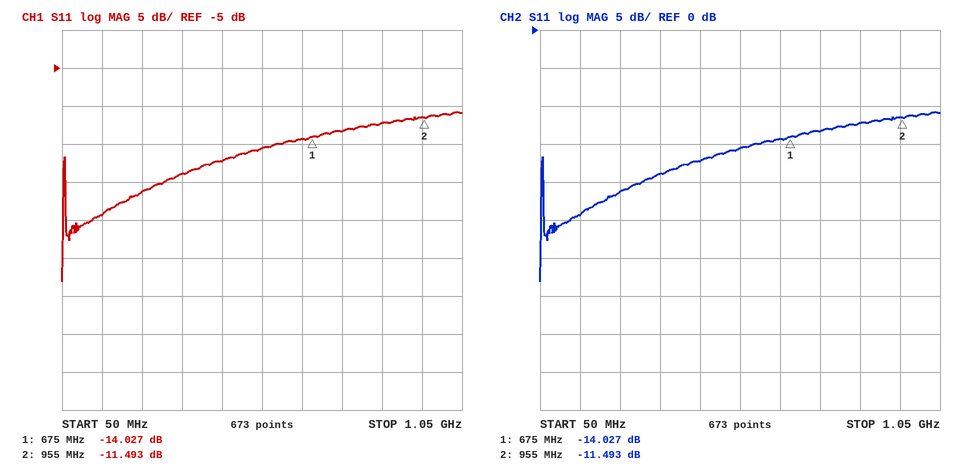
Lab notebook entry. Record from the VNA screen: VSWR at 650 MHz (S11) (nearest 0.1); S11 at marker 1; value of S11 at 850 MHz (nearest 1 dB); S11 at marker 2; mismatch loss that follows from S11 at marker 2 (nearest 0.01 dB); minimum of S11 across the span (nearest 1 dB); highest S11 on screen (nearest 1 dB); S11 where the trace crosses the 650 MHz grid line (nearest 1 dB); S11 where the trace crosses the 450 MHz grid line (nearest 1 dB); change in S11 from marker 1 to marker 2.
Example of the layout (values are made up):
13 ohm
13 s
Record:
1.5
-14.027 dB
-12 dB
-11.493 dB
0.32 dB
-33 dB
-11 dB
-14 dB
-17 dB
2.534 dB
